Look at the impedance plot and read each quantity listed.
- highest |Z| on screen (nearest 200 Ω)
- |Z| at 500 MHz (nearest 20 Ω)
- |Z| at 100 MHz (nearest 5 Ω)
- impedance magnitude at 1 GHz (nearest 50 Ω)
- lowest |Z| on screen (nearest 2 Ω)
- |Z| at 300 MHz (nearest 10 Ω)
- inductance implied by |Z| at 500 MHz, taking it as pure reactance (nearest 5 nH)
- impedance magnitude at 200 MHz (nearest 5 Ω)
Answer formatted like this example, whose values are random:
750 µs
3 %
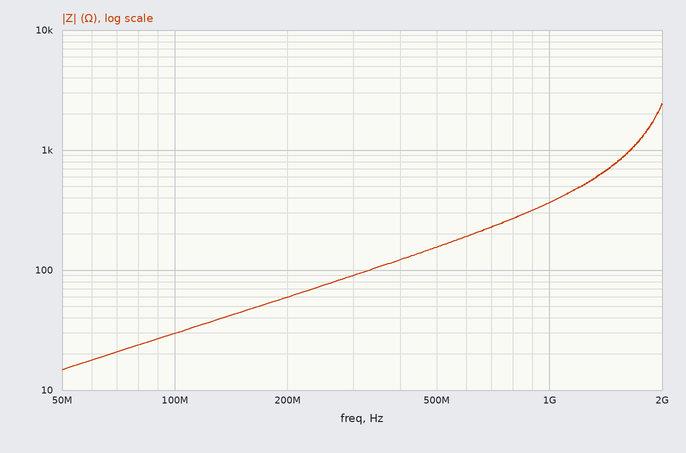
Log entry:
2.4 kΩ
160 Ω
30 Ω
350 Ω
14 Ω
90 Ω
50 nH
60 Ω
